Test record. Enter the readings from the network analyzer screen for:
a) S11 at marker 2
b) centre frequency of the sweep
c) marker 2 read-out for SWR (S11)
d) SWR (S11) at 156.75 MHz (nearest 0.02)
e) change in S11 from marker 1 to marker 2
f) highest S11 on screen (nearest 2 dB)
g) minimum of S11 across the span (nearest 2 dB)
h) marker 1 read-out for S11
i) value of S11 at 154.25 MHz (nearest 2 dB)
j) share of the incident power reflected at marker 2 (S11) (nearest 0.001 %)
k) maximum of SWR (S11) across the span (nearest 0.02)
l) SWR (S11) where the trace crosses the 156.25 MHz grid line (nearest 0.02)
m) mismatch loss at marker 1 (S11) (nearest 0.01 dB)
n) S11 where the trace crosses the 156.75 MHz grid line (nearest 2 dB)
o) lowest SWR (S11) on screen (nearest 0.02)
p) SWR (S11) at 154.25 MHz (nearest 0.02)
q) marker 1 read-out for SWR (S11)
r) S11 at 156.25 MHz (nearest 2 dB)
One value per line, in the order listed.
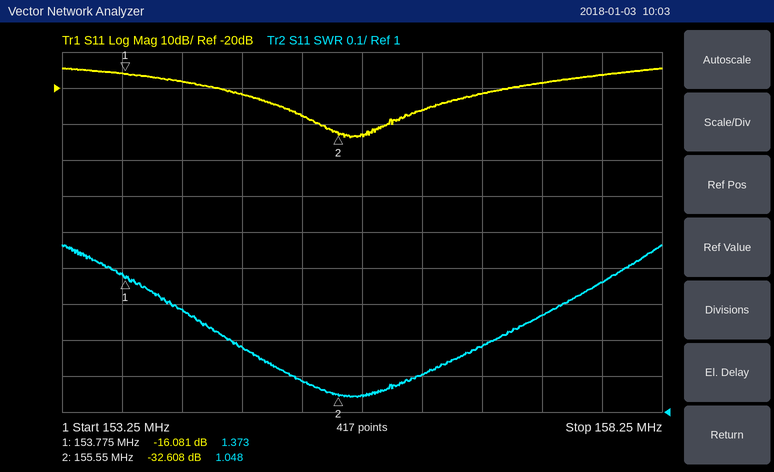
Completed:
-32.608 dB
155.75 MHz
1.048
1.18
-16.527 dB
-14 dB
-34 dB
-16.081 dB
-18 dB
0.055 %
1.46
1.10
0.11 dB
-22 dB
1.04
1.28
1.373
-26 dB
